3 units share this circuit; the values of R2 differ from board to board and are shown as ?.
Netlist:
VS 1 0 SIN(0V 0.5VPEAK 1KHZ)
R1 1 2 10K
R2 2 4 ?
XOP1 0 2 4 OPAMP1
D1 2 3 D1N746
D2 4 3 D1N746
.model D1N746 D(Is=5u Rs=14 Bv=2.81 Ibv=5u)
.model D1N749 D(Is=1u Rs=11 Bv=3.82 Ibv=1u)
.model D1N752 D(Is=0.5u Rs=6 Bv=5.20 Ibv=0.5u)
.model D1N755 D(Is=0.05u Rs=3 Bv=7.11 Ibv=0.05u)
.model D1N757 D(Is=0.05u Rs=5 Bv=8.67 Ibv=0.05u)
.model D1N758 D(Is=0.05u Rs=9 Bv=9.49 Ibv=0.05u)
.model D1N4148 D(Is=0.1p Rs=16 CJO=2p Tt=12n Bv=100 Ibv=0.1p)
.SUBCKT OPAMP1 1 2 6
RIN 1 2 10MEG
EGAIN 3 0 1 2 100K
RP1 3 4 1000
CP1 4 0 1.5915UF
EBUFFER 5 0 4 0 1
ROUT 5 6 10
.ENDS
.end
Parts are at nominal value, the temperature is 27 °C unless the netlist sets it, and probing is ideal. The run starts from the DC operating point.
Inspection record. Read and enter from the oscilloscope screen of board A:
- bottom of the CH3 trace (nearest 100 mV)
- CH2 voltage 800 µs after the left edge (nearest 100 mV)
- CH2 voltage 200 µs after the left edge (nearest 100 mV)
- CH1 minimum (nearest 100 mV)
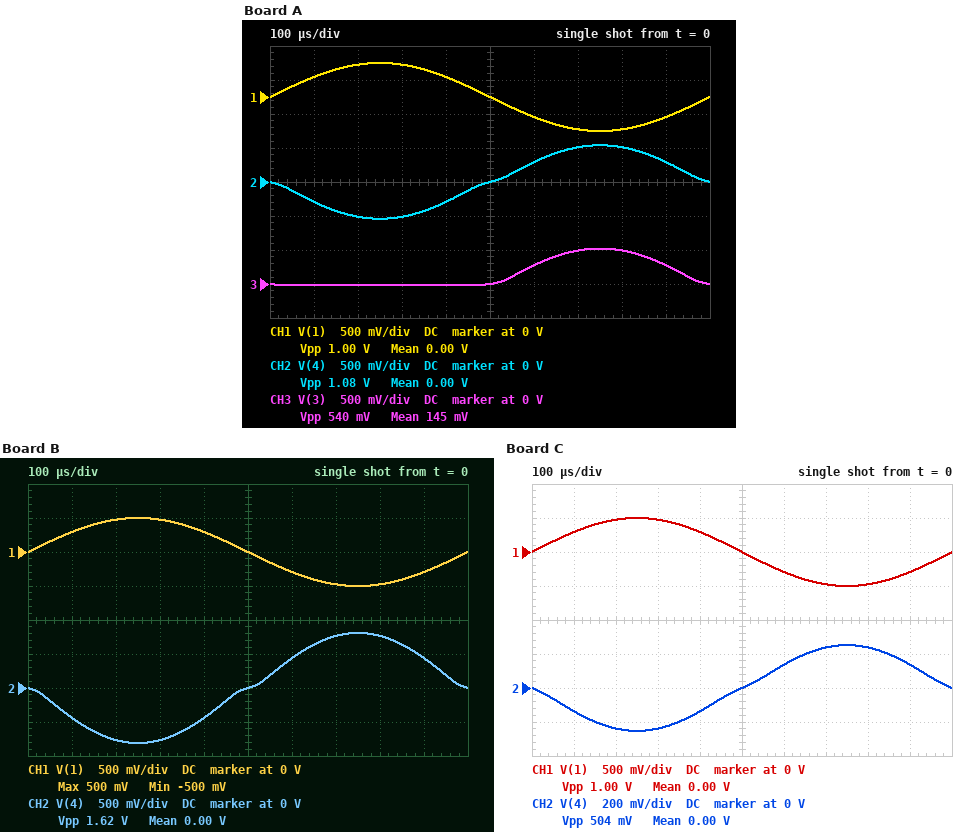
0 V
500 mV
-500 mV
-500 mV
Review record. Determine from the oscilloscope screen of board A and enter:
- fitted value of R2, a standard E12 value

12 kΩ
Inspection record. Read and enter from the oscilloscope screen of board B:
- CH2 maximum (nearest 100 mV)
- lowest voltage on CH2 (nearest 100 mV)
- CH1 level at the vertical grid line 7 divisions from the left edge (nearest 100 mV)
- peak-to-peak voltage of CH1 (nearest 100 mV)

800 mV
-800 mV
-500 mV
1.0 V
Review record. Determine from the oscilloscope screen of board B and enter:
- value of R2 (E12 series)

18 kΩ
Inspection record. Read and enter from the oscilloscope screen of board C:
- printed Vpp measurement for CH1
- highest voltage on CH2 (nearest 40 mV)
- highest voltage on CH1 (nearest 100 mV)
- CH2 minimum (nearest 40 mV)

1.00 V
240 mV
500 mV
-240 mV
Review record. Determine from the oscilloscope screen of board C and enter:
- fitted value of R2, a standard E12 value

5.6 kΩ
